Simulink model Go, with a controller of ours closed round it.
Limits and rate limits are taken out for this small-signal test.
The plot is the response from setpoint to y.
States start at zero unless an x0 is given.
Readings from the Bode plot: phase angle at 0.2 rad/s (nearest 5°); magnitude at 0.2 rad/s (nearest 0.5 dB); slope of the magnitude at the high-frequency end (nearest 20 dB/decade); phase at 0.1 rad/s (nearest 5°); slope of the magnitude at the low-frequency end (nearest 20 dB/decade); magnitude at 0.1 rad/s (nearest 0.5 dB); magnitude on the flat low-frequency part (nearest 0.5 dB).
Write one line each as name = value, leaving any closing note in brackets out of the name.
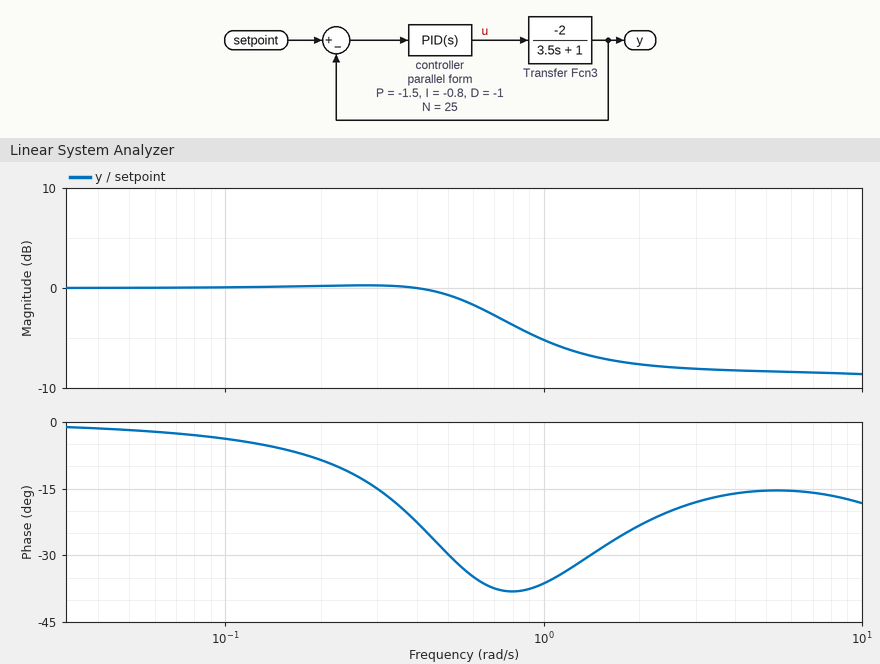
phase angle at 0.2 rad/s = -10°
magnitude at 0.2 rad/s = 0.0 dB
slope of the magnitude at the high-frequency end = 0 dB/decade
phase at 0.1 rad/s = -5°
slope of the magnitude at the low-frequency end = 0 dB/decade
magnitude at 0.1 rad/s = 0.0 dB
magnitude on the flat low-frequency part = 0.0 dB
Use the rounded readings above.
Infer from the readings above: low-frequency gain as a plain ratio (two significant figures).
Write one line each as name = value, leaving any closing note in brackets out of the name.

low-frequency gain as a plain ratio = 1.0
